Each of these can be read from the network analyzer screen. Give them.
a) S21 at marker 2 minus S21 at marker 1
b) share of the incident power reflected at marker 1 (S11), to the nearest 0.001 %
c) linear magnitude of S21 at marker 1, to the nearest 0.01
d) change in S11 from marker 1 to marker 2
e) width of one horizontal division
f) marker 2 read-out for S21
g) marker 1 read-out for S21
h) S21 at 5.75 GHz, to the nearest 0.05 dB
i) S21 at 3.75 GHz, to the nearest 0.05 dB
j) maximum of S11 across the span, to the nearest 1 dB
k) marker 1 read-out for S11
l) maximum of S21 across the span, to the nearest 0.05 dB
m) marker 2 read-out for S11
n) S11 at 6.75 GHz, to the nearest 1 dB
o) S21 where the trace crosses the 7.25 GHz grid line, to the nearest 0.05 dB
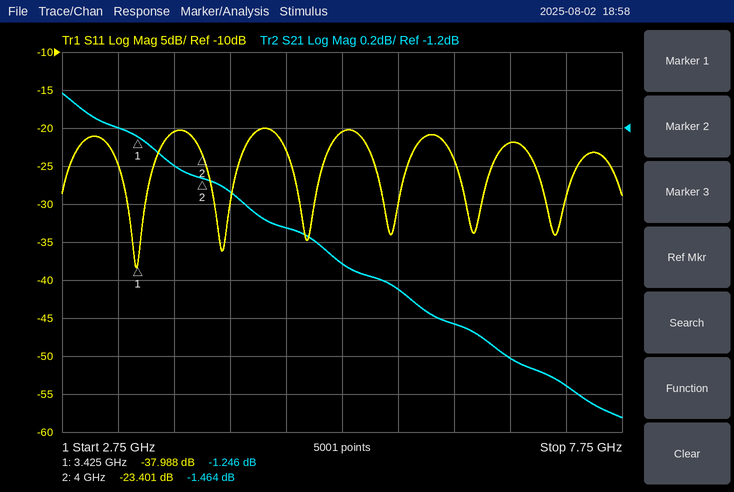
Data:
-0.218 dB
0.016 %
0.87
14.587 dB
500 MHz
-1.464 dB
-1.246 dB
-2.05 dB
-1.40 dB
-20 dB
-37.988 dB
-1.00 dB
-23.401 dB
-22 dB
-2.55 dB
